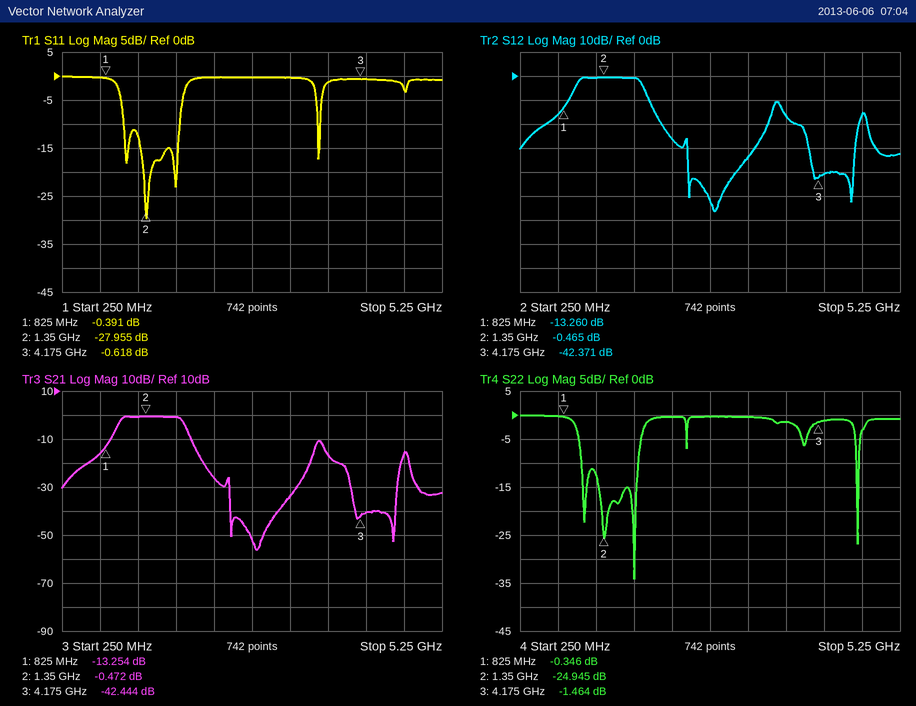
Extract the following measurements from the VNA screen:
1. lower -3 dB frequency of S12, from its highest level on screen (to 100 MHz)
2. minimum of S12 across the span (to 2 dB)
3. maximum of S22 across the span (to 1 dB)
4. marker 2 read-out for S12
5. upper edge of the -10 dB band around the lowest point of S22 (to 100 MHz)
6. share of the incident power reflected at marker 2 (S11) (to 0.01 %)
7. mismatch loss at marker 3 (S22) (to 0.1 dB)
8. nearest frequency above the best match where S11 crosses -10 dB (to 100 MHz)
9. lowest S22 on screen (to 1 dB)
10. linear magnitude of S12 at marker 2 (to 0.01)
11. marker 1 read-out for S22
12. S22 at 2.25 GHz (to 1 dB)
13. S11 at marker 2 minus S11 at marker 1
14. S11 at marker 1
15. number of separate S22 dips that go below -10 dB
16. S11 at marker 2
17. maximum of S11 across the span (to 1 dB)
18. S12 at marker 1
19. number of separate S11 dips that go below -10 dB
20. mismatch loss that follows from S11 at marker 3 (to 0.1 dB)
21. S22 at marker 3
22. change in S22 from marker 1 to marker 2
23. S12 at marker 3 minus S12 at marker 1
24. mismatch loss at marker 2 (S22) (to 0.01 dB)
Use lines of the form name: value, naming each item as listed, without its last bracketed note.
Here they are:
lower -3 dB frequency of S12, from its highest level on screen: 1.0 GHz
minimum of S12 across the span: -56 dB
maximum of S22 across the span: 0 dB
marker 2 read-out for S12: -0.465 dB
upper edge of the -10 dB band around the lowest point of S22: 1.8 GHz
share of the incident power reflected at marker 2 (S11): 0.16 %
mismatch loss at marker 3 (S22): 5.4 dB
nearest frequency above the best match where S11 crosses -10 dB: 1.8 GHz
lowest S22 on screen: -34 dB
linear magnitude of S12 at marker 2: 0.95
marker 1 read-out for S22: -0.346 dB
S22 at 2.25 GHz: 0 dB
S11 at marker 2 minus S11 at marker 1: -27.564 dB
S11 at marker 1: -0.391 dB
number of separate S22 dips that go below -10 dB: 4
S11 at marker 2: -27.955 dB
maximum of S11 across the span: 0 dB
S12 at marker 1: -13.260 dB
number of separate S11 dips that go below -10 dB: 4
mismatch loss that follows from S11 at marker 3: 8.8 dB
S22 at marker 3: -1.464 dB
change in S22 from marker 1 to marker 2: -24.599 dB
S12 at marker 3 minus S12 at marker 1: -29.111 dB
mismatch loss at marker 2 (S22): 0.01 dB
